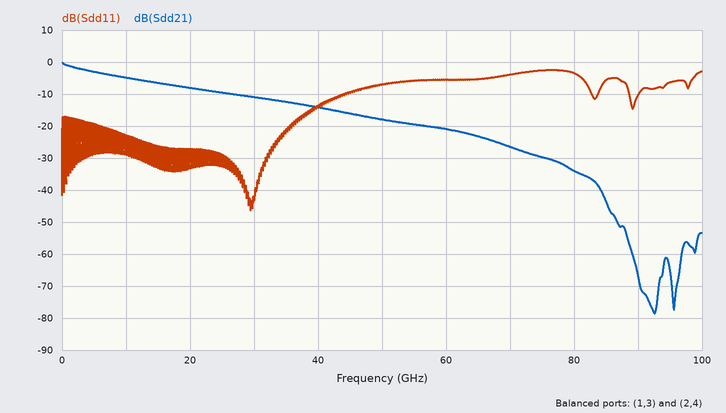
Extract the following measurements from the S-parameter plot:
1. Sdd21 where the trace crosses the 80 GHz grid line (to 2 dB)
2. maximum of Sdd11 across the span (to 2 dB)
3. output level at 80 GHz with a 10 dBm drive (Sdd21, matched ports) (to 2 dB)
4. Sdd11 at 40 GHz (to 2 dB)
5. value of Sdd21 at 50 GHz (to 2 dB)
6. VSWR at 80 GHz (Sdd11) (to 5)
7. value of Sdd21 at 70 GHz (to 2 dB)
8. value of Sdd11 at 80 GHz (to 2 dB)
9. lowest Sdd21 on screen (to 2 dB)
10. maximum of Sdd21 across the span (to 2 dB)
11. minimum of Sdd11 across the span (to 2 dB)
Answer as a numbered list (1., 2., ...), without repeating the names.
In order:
1. -34 dB
2. -2 dB
3. -24 dBm
4. -14 dB
5. -18 dB
6. 5
7. -26 dB
8. -4 dB
9. -78 dB
10. 0 dB
11. -46 dB
